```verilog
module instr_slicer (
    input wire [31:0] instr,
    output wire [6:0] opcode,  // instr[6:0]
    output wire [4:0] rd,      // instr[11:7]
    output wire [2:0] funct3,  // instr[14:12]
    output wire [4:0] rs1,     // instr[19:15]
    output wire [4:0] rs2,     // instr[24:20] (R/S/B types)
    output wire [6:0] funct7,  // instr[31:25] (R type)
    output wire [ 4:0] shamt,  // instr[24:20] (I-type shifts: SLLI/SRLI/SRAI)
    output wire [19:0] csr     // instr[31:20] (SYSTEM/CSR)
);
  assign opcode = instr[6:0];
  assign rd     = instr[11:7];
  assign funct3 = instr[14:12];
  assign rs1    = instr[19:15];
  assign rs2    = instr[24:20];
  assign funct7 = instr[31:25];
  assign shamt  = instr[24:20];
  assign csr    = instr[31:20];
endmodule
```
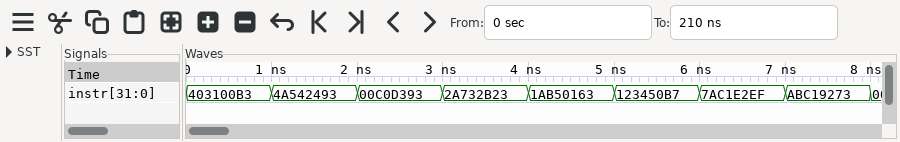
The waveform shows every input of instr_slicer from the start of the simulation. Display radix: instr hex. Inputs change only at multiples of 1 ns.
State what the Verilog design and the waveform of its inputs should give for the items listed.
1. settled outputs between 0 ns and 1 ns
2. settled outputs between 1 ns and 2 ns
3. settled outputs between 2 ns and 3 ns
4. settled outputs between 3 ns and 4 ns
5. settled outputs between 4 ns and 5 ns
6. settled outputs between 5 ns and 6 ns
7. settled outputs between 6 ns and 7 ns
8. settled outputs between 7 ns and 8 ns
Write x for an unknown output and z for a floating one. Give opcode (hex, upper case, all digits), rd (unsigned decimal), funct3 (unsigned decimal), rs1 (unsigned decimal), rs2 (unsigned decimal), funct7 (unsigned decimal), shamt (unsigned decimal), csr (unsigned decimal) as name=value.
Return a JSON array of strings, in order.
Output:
["opcode=33, rd=1, funct3=0, rs1=2, rs2=3, funct7=32, shamt=3, csr=1027", "opcode=13, rd=9, funct3=2, rs1=8, rs2=5, funct7=37, shamt=5, csr=1189", "opcode=13, rd=7, funct3=5, rs1=1, rs2=12, funct7=0, shamt=12, csr=12", "opcode=23, rd=22, funct3=2, rs1=6, rs2=7, funct7=21, shamt=7, csr=679", "opcode=63, rd=2, funct3=0, rs1=10, rs2=11, funct7=13, shamt=11, csr=427", "opcode=37, rd=1, funct3=5, rs1=8, rs2=3, funct7=9, shamt=3, csr=291", "opcode=6F, rd=5, funct3=6, rs1=3, rs2=12, funct7=61, shamt=12, csr=1964", "opcode=73, rd=4, funct3=1, rs1=3, rs2=28, funct7=85, shamt=28, csr=2748"]
